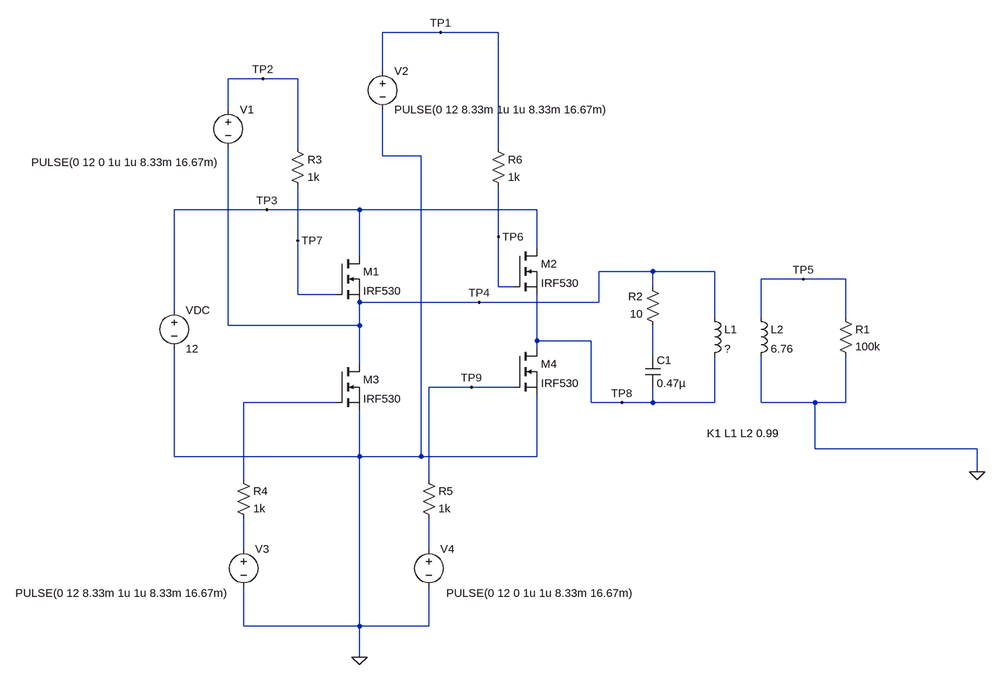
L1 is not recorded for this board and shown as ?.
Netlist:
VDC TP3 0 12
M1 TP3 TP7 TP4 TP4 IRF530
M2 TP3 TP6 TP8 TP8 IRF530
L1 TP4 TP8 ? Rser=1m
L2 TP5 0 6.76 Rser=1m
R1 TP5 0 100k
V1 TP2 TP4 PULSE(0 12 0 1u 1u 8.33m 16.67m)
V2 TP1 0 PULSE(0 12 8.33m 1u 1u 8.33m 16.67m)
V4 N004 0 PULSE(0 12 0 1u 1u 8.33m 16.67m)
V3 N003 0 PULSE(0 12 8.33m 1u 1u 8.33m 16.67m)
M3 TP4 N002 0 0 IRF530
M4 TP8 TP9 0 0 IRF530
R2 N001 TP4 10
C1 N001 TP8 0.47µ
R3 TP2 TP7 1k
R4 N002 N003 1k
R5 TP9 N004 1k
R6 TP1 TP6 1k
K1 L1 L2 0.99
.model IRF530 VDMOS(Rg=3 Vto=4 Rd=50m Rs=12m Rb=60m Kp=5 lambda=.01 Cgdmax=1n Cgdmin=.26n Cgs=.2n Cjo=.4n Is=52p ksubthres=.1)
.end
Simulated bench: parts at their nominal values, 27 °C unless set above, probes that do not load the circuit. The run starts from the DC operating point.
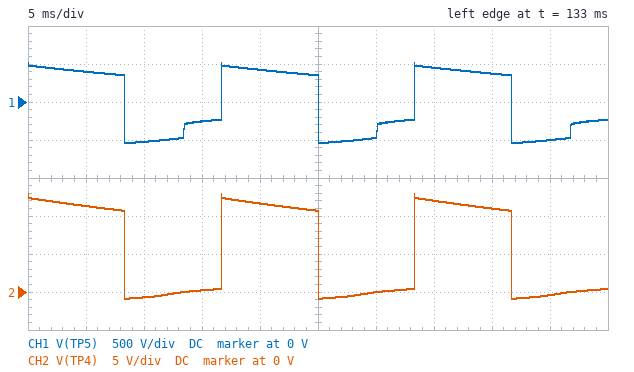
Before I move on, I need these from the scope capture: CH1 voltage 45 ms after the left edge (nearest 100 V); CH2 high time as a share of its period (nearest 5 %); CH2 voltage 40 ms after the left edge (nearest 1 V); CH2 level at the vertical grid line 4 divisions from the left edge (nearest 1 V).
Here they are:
-500 V
50 %
11 V
12 V
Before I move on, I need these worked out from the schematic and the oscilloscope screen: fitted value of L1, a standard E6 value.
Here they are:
4.7 mH
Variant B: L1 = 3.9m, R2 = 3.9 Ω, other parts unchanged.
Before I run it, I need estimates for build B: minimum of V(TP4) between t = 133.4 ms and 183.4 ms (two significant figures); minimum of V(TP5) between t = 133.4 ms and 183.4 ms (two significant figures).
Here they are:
-990 mV
-610 V
